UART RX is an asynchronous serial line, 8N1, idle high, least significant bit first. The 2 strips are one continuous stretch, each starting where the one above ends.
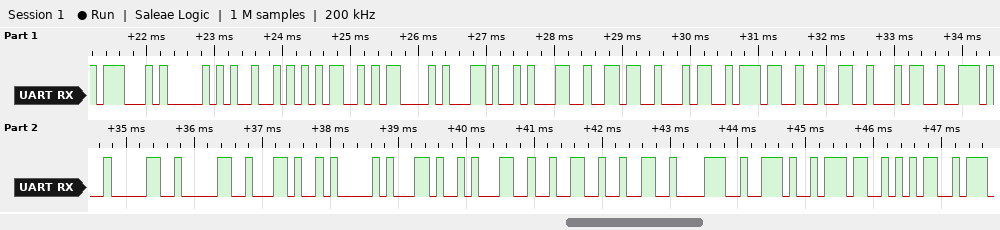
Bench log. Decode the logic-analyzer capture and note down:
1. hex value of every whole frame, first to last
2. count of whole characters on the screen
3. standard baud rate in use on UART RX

47 50 52 4D 43 2C 31 36 34 37 32 34 2E 30 30 2C 41 2C 31 32 32 38 2E 37 35
25
9600 baud
